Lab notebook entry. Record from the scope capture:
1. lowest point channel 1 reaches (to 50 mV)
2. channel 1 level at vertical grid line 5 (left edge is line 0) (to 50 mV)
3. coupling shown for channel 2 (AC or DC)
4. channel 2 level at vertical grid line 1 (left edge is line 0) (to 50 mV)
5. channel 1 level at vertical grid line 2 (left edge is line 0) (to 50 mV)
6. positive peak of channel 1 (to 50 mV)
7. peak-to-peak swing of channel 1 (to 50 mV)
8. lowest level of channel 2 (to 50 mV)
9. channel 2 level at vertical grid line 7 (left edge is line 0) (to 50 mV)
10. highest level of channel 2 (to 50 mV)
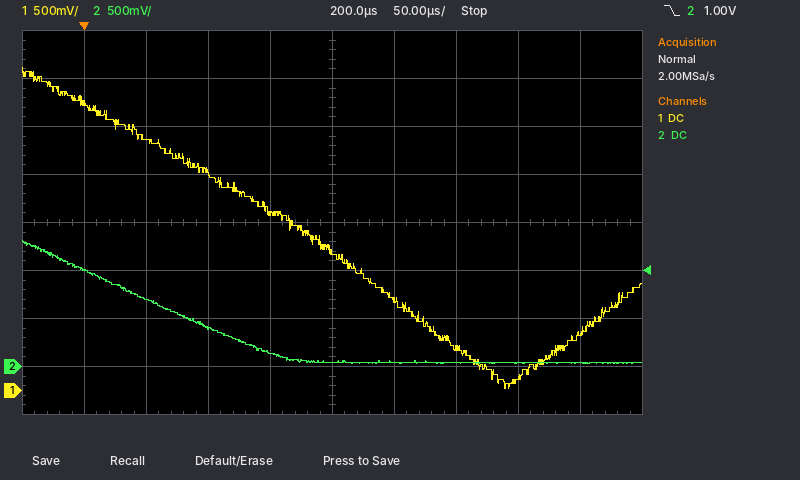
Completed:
0 mV
1.45 V
DC
1.00 V
2.60 V
3.35 V
3.35 V
50 mV
50 mV
1.30 V
